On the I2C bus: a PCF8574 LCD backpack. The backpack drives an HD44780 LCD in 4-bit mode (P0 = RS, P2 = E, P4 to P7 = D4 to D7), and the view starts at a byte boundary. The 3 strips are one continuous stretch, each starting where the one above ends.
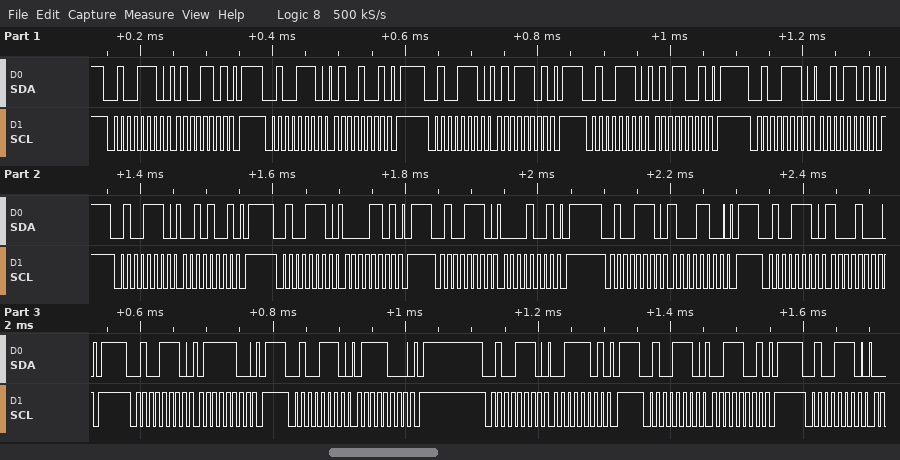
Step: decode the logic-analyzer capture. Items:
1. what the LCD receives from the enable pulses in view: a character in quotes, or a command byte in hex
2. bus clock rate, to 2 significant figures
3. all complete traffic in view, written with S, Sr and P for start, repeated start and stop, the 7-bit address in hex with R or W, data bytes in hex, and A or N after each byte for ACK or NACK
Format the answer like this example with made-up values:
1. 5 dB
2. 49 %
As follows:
1. 'E' ' ' 0x87
2. 100 kHz
3. S 27W A 4D A P S 27W A 49 A P S 27W A 5D A P S 27W A 59 A P S 27W A 2D A P S 27W A 29 A P S 27W A 0D A P S 27W A 09 A P S 27W A 8C A P S 27W A 88 A P S 27W A 7C A P S 27W A 78 A P S 27W A 3D A P S 27W A 39 A P S 27W A
